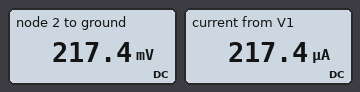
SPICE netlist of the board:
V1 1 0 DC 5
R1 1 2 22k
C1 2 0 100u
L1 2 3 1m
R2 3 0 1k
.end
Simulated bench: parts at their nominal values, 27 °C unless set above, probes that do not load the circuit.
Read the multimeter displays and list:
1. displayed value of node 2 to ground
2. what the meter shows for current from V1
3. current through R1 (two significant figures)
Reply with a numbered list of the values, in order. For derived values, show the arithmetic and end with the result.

1. 217.4 mV
2. 217.4 µA
3. (5 V - 217.4 mV) / 22 kΩ = 220 µA
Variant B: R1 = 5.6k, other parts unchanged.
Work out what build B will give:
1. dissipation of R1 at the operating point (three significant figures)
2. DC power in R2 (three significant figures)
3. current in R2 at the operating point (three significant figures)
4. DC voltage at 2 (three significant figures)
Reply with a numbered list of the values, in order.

1. 3.21 mW
2. 574 µW
3. 758 µA
4. 758 mV
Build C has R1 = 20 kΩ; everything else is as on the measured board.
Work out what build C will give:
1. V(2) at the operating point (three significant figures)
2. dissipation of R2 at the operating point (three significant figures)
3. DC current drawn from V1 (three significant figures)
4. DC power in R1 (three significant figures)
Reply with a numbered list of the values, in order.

1. 238 mV
2. 56.7 µW
3. 238 µA
4. 1.13 mW
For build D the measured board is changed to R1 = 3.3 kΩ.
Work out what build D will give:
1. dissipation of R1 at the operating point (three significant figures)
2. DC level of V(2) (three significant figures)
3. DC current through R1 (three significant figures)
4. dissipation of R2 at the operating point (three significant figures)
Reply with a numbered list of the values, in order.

1. 4.46 mW
2. 1.16 V
3. 1.16 mA
4. 1.35 mW
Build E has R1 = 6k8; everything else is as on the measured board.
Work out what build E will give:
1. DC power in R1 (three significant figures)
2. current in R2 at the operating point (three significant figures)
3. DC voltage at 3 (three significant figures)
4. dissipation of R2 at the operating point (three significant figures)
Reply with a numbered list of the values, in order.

1. 2.79 mW
2. 641 µA
3. 641 mV
4. 411 µW
